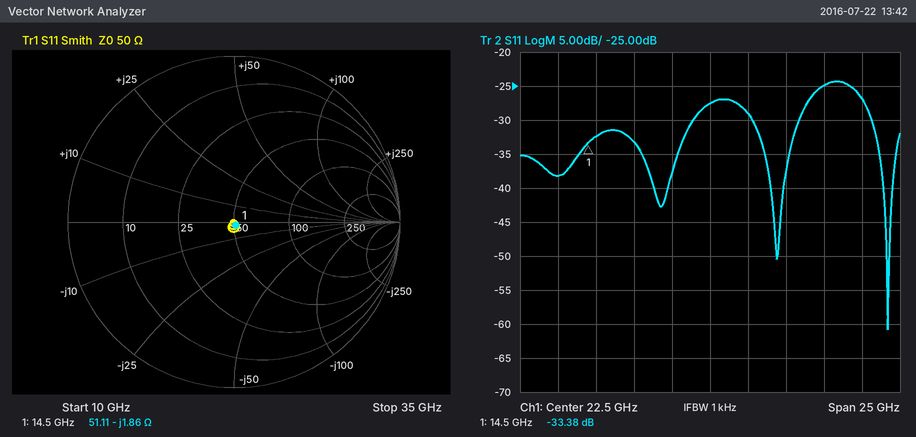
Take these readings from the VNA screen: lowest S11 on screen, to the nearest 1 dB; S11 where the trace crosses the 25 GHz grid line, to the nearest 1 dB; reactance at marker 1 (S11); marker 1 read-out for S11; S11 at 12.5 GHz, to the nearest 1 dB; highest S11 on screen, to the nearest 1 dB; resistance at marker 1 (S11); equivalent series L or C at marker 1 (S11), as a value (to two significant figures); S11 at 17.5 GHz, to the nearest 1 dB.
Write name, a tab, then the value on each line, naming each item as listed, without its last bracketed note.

lowest S11 on screen, to the nearest 1 dB	-61 dB
S11 where the trace crosses the 25 GHz grid line, to the nearest 1 dB	-29 dB
reactance at marker 1	-1.86 Ω
marker 1 read-out for S11	-33.38 dB
S11 at 12.5 GHz, to the nearest 1 dB	-38 dB
highest S11 on screen, to the nearest 1 dB	-24 dB
resistance at marker 1	51.11 Ω
equivalent series L or C at marker 1 (S11), as a value	5.9 pF
S11 at 17.5 GHz, to the nearest 1 dB	-33 dB
